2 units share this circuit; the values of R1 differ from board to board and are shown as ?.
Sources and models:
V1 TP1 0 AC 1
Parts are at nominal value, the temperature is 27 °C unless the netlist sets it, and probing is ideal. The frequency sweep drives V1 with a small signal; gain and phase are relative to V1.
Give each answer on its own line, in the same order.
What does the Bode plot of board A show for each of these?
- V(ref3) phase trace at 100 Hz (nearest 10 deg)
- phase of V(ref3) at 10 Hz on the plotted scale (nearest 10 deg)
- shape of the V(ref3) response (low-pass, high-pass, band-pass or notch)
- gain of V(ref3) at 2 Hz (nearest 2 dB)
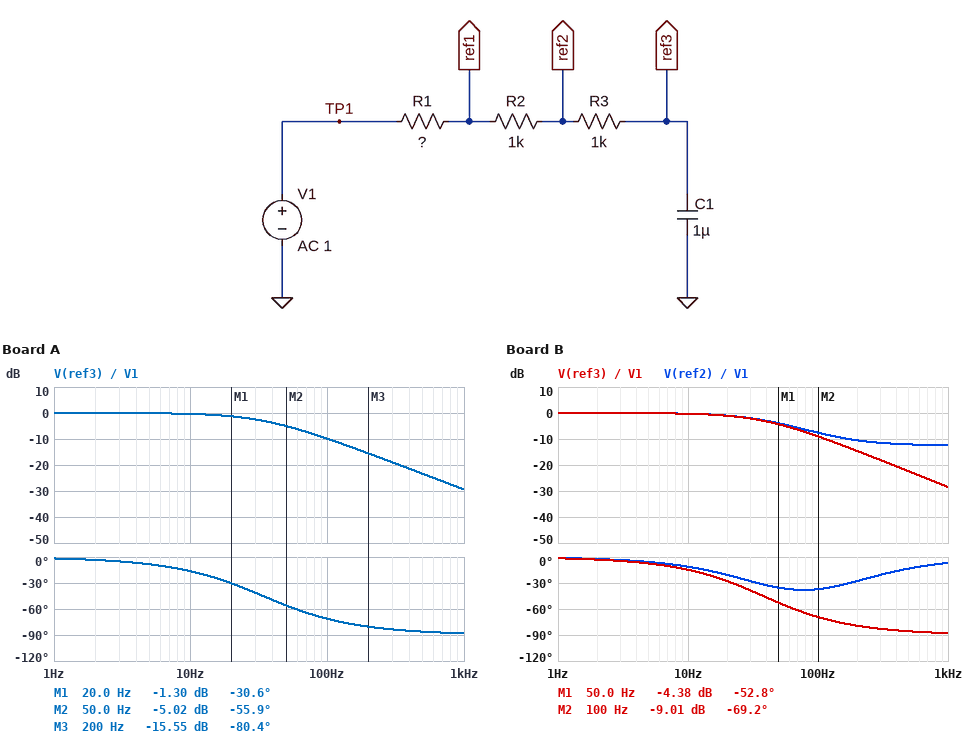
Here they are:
-70 deg
-20 deg
low-pass
0 dB
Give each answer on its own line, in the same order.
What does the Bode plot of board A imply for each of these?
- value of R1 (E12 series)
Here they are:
2.7 kΩ
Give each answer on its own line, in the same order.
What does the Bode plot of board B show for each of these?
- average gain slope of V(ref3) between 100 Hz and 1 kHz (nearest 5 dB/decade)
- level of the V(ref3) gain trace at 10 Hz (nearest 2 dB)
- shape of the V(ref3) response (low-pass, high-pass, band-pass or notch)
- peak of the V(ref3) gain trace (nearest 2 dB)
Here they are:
-20 dB/decade
0 dB
low-pass
0 dB
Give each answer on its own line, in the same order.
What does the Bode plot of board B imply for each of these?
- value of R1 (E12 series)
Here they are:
2.2 kΩ
